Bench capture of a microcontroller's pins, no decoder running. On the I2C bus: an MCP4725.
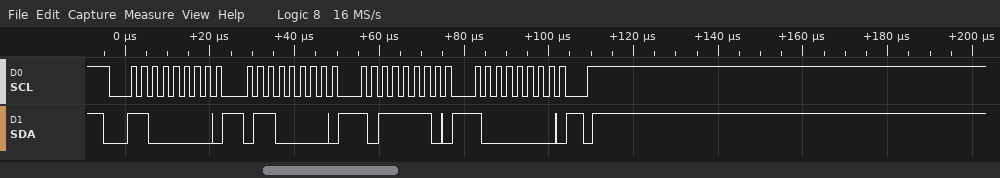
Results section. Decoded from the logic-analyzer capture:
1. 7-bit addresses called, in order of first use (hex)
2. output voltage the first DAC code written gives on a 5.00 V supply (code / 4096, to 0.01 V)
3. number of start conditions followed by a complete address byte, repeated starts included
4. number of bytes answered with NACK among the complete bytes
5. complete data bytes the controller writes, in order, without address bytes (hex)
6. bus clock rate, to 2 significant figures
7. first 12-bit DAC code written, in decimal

0x60
3.72 V
1
0
60 BE 80
400 kHz
3048
